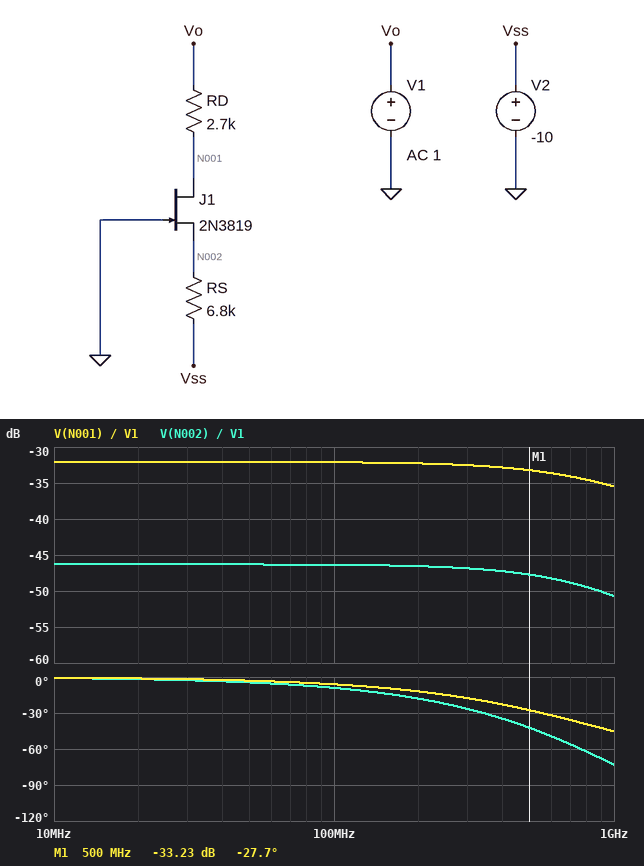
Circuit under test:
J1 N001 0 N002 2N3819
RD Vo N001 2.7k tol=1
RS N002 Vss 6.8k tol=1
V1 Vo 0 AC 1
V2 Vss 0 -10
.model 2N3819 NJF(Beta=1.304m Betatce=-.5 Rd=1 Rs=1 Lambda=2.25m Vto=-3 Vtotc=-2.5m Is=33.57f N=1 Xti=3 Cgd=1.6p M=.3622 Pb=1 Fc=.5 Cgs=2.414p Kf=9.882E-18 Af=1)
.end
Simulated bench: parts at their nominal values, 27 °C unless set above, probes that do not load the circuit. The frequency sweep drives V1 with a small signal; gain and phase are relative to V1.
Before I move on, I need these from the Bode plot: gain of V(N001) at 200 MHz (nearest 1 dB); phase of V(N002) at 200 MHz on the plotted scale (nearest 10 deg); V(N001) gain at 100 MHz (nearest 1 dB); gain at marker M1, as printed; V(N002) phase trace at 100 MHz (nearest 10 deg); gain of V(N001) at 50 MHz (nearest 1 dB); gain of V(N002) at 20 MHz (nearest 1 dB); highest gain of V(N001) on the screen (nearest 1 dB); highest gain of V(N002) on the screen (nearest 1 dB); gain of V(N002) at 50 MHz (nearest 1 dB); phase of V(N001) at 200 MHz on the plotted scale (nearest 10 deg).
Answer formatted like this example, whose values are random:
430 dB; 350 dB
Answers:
-32 dB; -20 deg; -32 dB; -33.23 dB; -10 deg; -32 dB; -46 dB; -32 dB; -46 dB; -46 dB; -10 deg
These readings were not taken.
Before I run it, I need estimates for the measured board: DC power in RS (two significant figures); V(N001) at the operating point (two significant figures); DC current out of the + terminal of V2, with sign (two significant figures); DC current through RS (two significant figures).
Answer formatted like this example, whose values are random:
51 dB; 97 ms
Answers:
13 mW; -580 mV; -1.4 mA; 1.4 mA
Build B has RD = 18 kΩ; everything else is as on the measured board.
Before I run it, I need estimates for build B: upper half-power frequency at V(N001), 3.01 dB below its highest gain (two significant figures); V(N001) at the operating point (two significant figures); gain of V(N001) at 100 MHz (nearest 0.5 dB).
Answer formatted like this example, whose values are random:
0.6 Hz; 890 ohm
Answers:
1.1 GHz; -590 mV; -50.5 dB
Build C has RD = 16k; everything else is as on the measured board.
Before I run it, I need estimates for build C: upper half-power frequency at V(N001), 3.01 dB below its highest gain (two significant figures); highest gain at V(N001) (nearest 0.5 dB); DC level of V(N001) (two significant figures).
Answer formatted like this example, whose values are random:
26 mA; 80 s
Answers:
1.1 GHz; -49.5 dB; -590 mV
